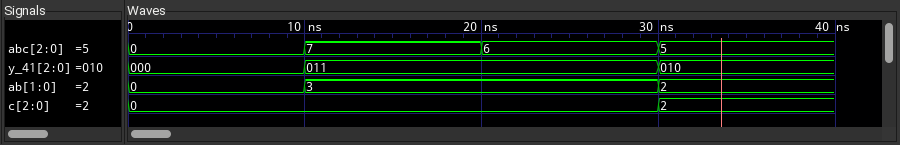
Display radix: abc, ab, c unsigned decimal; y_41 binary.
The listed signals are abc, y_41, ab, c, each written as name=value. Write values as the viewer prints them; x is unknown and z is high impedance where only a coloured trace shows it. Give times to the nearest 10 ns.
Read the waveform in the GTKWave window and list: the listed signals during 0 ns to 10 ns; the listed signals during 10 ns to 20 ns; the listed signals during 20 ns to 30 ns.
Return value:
abc=0, y_41=000, ab=0, c=0
abc=7, y_41=011, ab=3, c=0
abc=6, y_41=011, ab=3, c=0
